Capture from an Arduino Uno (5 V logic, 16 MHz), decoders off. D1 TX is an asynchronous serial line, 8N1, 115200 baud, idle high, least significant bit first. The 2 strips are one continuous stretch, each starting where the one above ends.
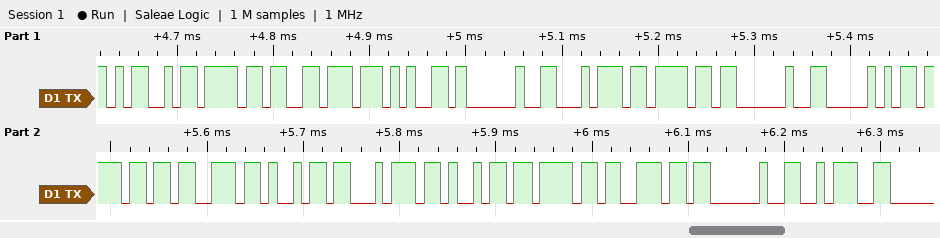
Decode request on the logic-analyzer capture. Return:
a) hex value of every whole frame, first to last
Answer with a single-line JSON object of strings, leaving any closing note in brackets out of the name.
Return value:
{"hex value of every whole frame, first to last": "4D 6F 76 65 20 74 6F 20 50 6F 73 69 74 69 6F 6E 20 3A"}
